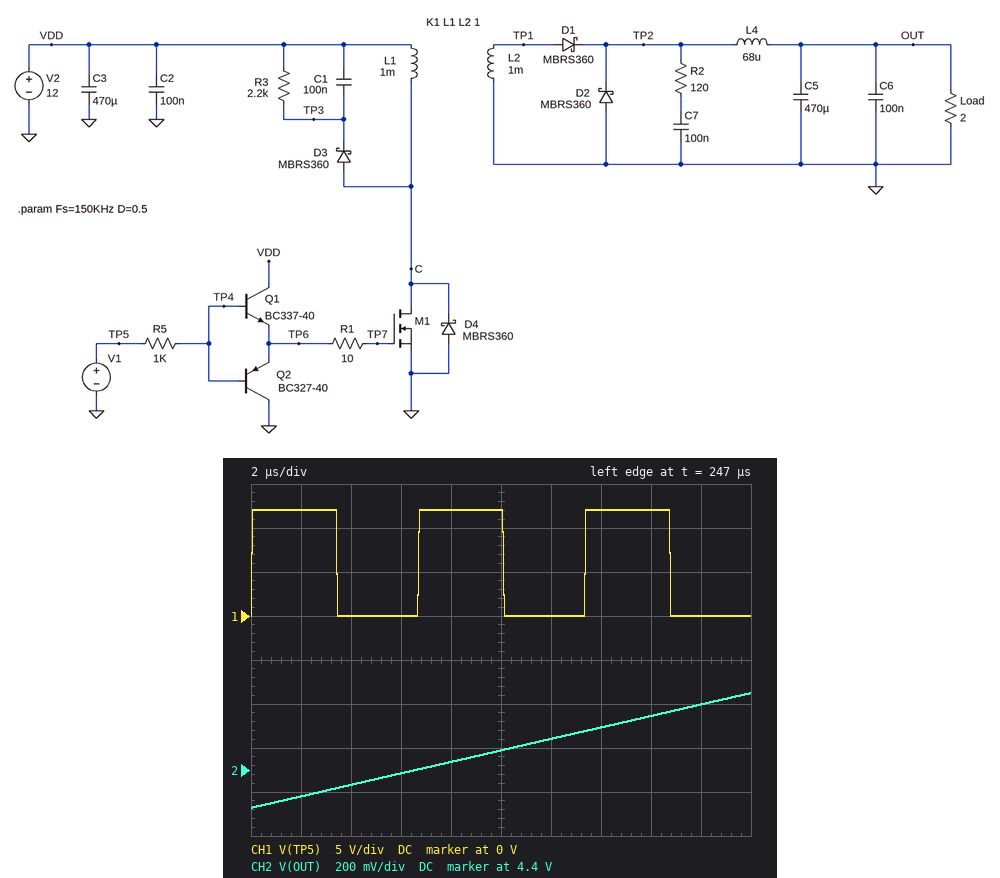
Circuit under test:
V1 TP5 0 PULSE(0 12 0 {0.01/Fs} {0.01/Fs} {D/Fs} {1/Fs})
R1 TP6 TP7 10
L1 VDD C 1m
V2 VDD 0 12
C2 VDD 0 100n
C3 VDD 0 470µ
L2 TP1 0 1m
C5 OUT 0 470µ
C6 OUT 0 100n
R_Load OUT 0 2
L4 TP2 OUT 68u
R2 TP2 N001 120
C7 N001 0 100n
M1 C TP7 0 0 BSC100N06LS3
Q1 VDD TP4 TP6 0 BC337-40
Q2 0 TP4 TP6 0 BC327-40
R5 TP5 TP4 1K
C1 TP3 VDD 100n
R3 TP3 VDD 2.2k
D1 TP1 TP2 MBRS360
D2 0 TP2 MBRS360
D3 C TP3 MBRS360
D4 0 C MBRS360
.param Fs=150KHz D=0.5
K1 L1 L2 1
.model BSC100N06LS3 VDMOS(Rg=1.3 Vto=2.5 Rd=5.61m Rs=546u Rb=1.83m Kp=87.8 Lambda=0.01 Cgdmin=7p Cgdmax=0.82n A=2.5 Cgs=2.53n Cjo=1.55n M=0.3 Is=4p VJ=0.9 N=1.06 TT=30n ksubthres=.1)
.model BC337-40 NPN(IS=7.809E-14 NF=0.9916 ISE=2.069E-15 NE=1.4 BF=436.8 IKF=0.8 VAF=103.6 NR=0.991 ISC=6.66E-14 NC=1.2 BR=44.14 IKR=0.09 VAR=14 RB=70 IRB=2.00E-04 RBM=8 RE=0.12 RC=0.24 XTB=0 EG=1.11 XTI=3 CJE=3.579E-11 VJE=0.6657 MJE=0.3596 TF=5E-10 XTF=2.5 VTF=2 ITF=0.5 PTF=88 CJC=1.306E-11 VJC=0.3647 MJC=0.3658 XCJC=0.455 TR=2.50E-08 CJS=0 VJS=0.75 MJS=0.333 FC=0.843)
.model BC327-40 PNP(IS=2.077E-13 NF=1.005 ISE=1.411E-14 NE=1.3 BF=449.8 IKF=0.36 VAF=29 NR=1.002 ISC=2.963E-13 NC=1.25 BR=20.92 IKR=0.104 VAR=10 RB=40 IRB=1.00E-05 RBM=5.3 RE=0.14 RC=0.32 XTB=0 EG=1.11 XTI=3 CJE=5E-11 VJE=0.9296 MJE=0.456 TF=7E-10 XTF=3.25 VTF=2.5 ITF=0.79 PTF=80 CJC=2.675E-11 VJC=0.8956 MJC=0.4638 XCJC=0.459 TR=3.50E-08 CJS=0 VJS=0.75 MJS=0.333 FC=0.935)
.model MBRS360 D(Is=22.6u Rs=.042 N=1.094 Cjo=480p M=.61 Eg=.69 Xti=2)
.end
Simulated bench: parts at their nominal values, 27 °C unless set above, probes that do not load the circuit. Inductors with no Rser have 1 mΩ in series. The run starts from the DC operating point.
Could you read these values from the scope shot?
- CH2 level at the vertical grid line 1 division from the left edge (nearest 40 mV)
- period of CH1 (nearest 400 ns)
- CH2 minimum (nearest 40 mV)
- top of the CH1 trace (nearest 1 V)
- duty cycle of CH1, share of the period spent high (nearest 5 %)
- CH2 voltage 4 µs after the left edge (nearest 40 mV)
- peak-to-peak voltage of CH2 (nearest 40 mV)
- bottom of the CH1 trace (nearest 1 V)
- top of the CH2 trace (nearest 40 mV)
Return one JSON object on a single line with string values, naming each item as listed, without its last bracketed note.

{"CH2 level at the vertical grid line 1 division from the left edge": "4.28 V", "period of CH1": "6.8 µs", "CH2 minimum": "4.24 V", "top of the CH1 trace": "12 V", "duty cycle of CH1, share of the period spent high": "50 %", "CH2 voltage 4 µs after the left edge": "4.32 V", "peak-to-peak voltage of CH2": "520 mV", "bottom of the CH1 trace": "0 V", "top of the CH2 trace": "4.76 V"}
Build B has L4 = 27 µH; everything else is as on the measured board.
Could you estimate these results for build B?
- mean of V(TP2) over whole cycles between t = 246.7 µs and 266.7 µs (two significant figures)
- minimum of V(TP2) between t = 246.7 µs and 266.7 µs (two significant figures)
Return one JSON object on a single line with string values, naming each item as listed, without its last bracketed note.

{"mean of V(TP2) over whole cycles between t = 246.7 µs and 266.7 µs": "5.1 V", "minimum of V(TP2) between t = 246.7 µs and 266.7 µs": "-1.1 V"}
